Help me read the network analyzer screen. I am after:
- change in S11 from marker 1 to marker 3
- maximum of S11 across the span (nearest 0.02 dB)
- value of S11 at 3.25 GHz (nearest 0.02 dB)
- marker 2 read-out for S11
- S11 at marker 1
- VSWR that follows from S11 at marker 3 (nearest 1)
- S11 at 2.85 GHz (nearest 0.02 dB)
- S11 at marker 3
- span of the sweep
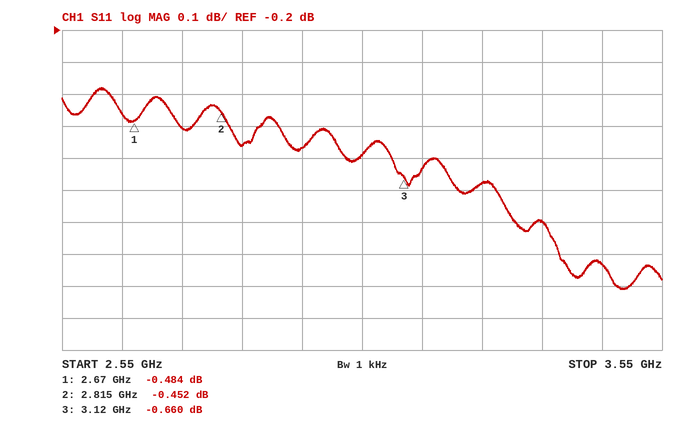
-0.176 dB
-0.38 dB
-0.68 dB
-0.452 dB
-0.484 dB
26
-0.56 dB
-0.660 dB
1 GHz
